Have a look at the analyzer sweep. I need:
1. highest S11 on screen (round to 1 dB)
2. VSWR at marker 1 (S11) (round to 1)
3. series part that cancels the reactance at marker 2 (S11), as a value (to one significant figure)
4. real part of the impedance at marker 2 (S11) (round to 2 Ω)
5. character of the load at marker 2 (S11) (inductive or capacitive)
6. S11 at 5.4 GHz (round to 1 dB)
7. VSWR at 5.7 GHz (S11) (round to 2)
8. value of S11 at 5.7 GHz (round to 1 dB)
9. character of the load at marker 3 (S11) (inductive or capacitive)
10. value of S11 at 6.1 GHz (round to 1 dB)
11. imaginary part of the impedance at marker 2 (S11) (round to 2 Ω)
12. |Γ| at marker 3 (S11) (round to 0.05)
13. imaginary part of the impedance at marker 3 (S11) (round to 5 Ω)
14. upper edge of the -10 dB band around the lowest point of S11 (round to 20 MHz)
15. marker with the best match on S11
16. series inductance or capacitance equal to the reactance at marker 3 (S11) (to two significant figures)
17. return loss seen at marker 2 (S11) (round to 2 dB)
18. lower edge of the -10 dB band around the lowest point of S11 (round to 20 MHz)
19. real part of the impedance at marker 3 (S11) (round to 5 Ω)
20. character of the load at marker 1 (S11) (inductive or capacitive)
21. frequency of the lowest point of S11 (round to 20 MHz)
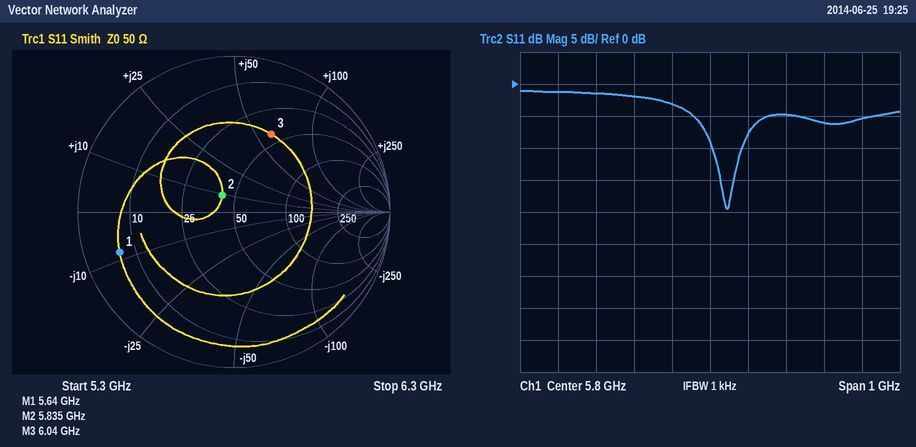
-1 dB
8
3 pF
42 Ω
inductive
-1 dB
6
-3 dB
inductive
-6 dB
+10 Ω
0.55
+60 Ω
5.88 GHz
marker 2
1.6 nH
18 dB
5.80 GHz
40 Ω
capacitive
5.84 GHz
